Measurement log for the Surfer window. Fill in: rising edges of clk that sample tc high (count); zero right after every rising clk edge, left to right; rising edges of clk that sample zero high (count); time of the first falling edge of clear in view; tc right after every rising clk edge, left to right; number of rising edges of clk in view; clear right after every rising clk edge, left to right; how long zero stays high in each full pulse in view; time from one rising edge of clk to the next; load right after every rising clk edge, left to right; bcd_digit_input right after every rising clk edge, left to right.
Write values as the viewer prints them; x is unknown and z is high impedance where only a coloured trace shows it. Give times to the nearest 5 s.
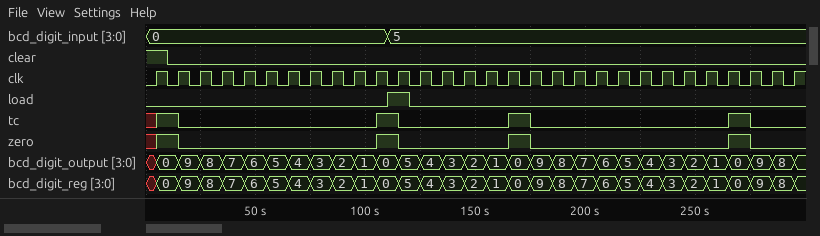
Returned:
4
1 0 0 0 0 0 0 0 0 0 1 0 0 0 0 0 1 0 0 0 0 0 0 0 0 0 1 0 0 0
4
10 s
1 0 0 0 0 0 0 0 0 0 1 0 0 0 0 0 1 0 0 0 0 0 0 0 0 0 1 0 0 0
30
1 0 0 0 0 0 0 0 0 0 0 0 0 0 0 0 0 0 0 0 0 0 0 0 0 0 0 0 0 0
10 s, 10 s, 10 s
10 s
0 0 0 0 0 0 0 0 0 0 0 1 0 0 0 0 0 0 0 0 0 0 0 0 0 0 0 0 0 0
0, 0, 0, 0, 0, 0, 0, 0, 0, 0, 0, 5, 5, 5, 5, 5, 5, 5, 5, 5, 5, 5, 5, 5, 5, 5, 5, 5, 5, 5
